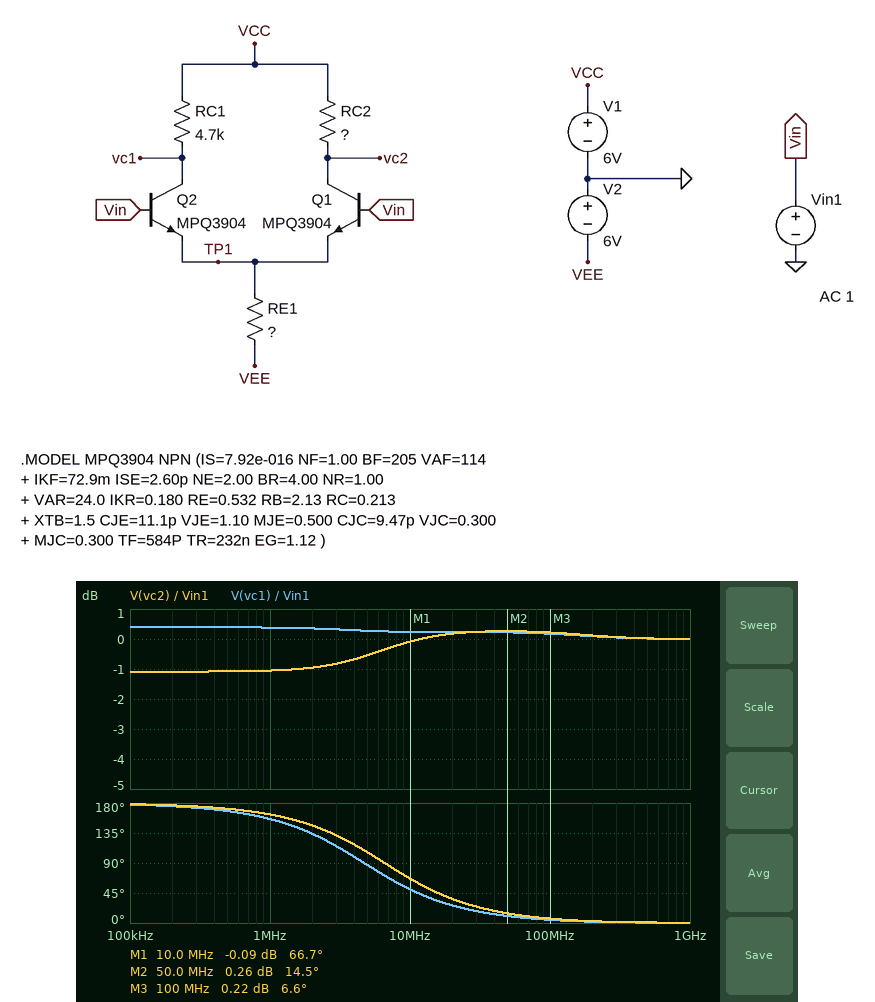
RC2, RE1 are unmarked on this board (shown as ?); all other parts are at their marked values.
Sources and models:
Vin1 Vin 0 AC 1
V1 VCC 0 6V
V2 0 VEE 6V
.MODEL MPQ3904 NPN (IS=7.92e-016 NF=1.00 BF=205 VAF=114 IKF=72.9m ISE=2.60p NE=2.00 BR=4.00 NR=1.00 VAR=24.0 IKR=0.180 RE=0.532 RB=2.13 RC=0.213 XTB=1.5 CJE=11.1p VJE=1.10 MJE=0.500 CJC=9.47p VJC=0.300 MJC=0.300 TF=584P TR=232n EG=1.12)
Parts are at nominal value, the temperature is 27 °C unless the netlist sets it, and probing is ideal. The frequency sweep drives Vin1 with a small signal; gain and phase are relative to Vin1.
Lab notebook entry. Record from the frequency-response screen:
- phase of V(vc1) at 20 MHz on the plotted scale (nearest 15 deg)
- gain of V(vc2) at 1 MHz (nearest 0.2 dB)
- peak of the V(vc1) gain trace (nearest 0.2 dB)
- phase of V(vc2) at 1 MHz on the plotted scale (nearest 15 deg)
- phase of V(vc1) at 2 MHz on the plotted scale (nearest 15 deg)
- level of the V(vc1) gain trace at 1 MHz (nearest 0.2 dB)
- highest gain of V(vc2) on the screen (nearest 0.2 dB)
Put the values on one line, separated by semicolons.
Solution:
30 deg; -1.0 dB; 0.4 dB; 165 deg; 135 deg; 0.4 dB; 0.2 dB
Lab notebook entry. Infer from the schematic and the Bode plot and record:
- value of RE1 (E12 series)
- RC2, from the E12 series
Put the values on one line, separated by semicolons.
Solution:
2.2 kΩ; 3.9 kΩ
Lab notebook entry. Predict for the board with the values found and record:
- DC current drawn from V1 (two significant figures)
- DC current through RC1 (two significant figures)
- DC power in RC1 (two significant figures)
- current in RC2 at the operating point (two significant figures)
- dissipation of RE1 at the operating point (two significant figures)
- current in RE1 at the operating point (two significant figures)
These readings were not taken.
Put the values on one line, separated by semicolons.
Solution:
2.4 mA; 1.2 mA; 6.6 mW; 1.2 mA; 13 mW; 2.4 mA
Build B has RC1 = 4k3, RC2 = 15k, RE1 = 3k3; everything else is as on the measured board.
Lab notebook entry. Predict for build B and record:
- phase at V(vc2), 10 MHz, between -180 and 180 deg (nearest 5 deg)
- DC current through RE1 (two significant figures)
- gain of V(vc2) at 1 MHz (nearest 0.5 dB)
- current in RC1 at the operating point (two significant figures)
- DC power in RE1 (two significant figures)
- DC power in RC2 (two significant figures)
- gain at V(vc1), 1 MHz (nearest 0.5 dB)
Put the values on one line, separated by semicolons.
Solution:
0 deg; 1.6 mA; 0 dB; 1.0 mA; 8.4 mW; 3.0 mW; -1.5 dB
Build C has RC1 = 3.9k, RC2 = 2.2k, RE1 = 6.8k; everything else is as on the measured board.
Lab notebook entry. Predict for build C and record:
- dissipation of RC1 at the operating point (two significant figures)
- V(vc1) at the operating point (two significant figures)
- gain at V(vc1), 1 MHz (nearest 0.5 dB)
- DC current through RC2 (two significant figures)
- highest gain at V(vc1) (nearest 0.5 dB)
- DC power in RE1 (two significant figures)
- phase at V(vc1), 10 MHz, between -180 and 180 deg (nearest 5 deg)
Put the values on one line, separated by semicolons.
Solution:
580 µW; 4.5 V; -10.5 dB; 390 µA; 0 dB; 4.1 mW; 60 deg
